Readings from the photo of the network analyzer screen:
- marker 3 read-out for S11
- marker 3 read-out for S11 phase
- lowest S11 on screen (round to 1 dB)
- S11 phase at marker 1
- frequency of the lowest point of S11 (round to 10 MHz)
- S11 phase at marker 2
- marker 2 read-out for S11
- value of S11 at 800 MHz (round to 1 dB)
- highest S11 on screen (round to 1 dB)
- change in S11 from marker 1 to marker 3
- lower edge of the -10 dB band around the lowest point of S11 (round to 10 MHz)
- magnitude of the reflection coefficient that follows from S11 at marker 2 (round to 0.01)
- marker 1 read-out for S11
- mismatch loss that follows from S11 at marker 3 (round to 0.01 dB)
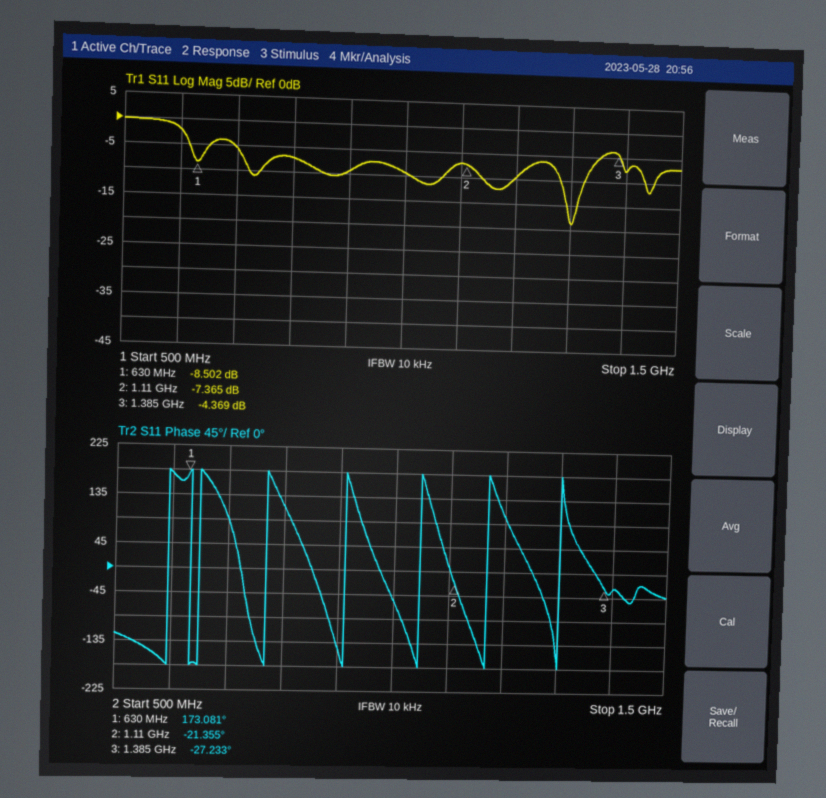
-4.369 dB
-27.233°
-19 dB
173.081°
1.30 GHz
-21.355°
-7.365 dB
-7 dB
0 dB
4.133 dB
1.28 GHz
0.43
-8.502 dB
1.98 dB
